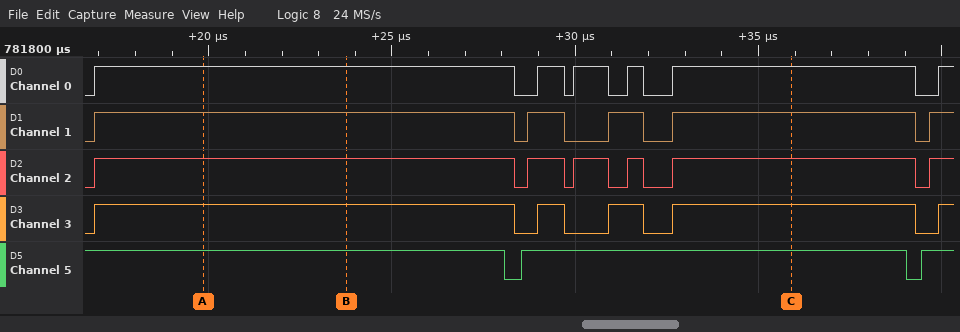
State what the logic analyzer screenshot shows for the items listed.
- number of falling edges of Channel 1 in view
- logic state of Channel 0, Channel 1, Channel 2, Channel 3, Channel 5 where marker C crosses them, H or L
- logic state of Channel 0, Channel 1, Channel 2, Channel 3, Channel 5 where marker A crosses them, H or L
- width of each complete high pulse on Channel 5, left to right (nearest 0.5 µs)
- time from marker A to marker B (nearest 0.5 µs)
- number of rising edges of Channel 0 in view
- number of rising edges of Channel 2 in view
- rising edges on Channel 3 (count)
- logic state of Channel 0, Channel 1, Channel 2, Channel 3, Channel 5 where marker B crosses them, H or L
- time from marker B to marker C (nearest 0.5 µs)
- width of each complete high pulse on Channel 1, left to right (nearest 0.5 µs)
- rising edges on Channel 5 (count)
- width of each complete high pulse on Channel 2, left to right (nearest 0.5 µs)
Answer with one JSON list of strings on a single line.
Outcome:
["4", "Channel 0=H, Channel 1=H, Channel 2=H, Channel 3=H, Channel 5=H", "Channel 0=H, Channel 1=H, Channel 2=H, Channel 3=H, Channel 5=H", "10.5 µs", "4 µs", "6", "6", "5", "Channel 0=H, Channel 1=H, Channel 2=H, Channel 3=H, Channel 5=H", "12 µs", "11.5 µs, 1 µs, 1 µs, 6.5 µs", "2", "11.5 µs, 1 µs, 1 µs, 0.5 µs, 6.5 µs"]
